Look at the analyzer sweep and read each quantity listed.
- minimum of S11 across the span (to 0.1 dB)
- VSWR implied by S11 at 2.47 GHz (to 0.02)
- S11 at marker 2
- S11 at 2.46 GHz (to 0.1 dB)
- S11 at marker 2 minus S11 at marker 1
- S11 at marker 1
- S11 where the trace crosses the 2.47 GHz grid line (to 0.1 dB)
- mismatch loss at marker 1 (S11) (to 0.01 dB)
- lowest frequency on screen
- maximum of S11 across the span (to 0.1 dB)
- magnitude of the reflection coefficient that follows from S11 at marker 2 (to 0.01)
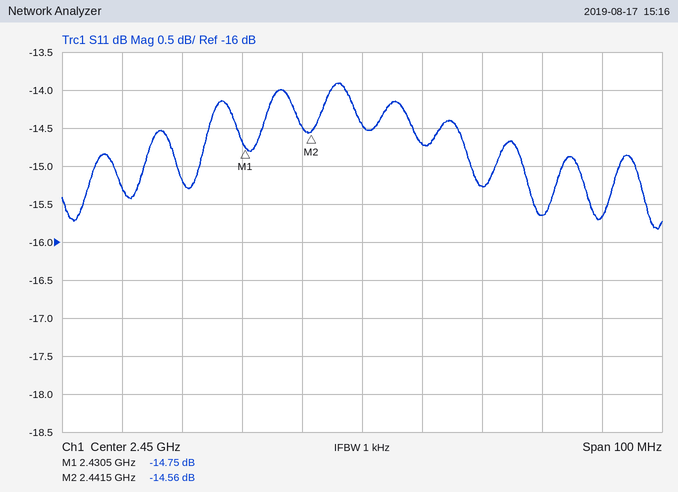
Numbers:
-15.8 dB
1.42
-14.56 dB
-14.7 dB
0.19 dB
-14.75 dB
-15.3 dB
0.15 dB
2.4 GHz
-13.9 dB
0.19
